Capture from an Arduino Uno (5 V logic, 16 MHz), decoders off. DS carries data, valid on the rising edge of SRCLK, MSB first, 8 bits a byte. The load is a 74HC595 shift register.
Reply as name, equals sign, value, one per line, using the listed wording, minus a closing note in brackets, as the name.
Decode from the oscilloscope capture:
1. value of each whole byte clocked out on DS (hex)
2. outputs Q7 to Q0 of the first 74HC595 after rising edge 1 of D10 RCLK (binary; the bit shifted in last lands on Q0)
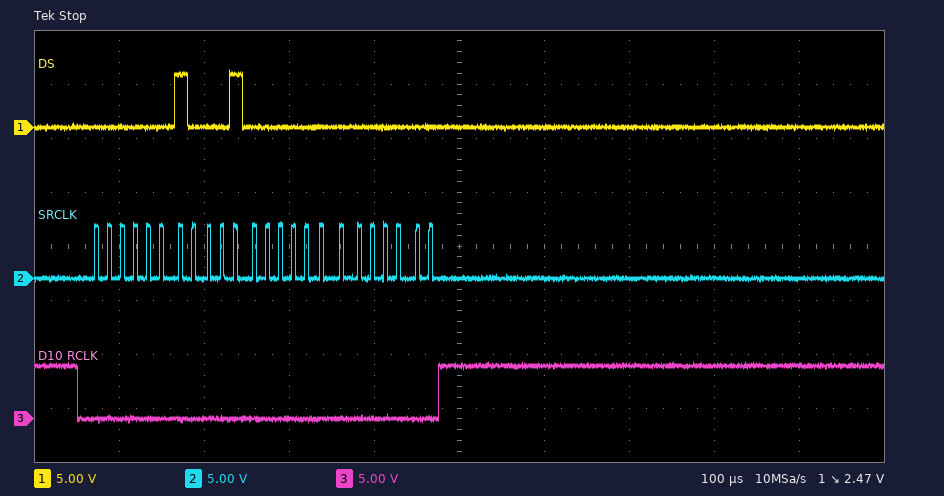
value of each whole byte clocked out on DS = 02 20 00
outputs Q7 to Q0 of the first 74HC595 after rising edge 1 of D10 RCLK = 00000000
